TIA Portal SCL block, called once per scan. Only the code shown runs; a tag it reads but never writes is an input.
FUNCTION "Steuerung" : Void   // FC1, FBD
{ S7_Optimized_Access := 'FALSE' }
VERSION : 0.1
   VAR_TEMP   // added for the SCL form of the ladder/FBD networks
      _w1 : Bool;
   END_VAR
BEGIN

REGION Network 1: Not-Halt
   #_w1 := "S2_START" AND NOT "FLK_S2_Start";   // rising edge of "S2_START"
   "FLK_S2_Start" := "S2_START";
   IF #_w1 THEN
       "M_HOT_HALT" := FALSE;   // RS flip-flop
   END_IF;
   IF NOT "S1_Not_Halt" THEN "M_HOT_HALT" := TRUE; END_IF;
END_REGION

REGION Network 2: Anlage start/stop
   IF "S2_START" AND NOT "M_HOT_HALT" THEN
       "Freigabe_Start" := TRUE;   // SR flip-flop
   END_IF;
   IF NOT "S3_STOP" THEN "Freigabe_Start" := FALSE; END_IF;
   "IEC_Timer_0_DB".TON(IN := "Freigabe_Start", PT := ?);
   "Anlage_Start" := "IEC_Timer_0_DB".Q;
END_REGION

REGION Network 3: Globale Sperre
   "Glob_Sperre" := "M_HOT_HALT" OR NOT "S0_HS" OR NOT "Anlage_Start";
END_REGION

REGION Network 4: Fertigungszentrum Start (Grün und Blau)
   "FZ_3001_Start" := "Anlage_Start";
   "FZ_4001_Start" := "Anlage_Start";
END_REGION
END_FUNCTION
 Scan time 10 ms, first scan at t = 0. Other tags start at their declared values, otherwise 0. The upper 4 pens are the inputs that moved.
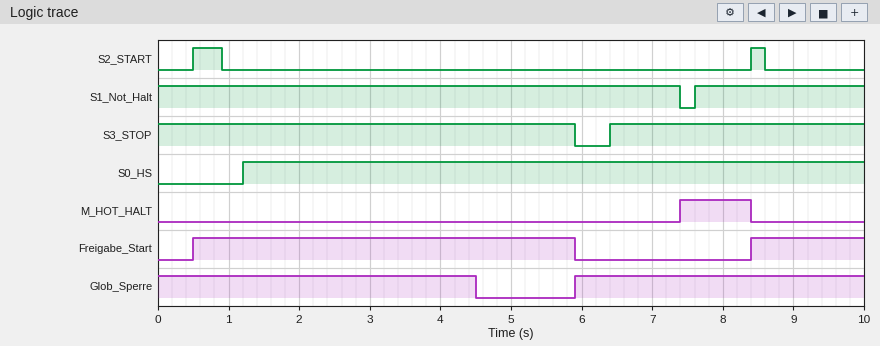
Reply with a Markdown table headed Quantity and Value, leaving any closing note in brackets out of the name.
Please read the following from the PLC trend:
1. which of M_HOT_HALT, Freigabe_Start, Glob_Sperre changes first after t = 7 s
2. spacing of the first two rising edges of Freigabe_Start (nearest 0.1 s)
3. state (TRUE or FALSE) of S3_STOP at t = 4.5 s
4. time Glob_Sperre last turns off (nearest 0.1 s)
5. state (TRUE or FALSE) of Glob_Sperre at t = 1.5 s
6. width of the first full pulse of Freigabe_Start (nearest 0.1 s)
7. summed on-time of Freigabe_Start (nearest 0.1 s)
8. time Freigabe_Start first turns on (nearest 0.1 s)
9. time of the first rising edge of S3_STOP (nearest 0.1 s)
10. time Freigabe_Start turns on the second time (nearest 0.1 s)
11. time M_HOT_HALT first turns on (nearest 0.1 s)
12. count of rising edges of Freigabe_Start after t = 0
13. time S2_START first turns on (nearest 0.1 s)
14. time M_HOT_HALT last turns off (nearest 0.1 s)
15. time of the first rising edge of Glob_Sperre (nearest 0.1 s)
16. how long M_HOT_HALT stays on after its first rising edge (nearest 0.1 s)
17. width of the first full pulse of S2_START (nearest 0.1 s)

| Quantity | Value |
|---|---|
| which of M_HOT_HALT, Freigabe_Start, Glob_Sperre changes first after t = 7 s | M_HOT_HALT |
| spacing of the first two rising edges of Freigabe_Start | 7.9 s |
| state (TRUE or FALSE) of S3_STOP at t = 4.5 s | TRUE |
| time Glob_Sperre last turns off | 4.5 s |
| state (TRUE or FALSE) of Glob_Sperre at t = 1.5 s | TRUE |
| width of the first full pulse of Freigabe_Start | 5.4 s |
| summed on-time of Freigabe_Start | 7.0 s |
| time Freigabe_Start first turns on | 0.5 s |
| time of the first rising edge of S3_STOP | 6.4 s |
| time Freigabe_Start turns on the second time | 8.4 s |
| time M_HOT_HALT first turns on | 7.4 s |
| count of rising edges of Freigabe_Start after t = 0 | 2 |
| time S2_START first turns on | 0.5 s |
| time M_HOT_HALT last turns off | 8.4 s |
| time of the first rising edge of Glob_Sperre | 5.9 s |
| how long M_HOT_HALT stays on after its first rising edge | 1.0 s |
| width of the first full pulse of S2_START | 0.4 s |
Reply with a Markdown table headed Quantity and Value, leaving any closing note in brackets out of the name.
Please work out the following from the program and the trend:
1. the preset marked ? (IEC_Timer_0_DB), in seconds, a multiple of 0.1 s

| Quantity | Value |
|---|---|
| the preset marked ? (IEC_Timer_0_DB), in seconds, a multiple of 0.1 s | 4.0 s |
